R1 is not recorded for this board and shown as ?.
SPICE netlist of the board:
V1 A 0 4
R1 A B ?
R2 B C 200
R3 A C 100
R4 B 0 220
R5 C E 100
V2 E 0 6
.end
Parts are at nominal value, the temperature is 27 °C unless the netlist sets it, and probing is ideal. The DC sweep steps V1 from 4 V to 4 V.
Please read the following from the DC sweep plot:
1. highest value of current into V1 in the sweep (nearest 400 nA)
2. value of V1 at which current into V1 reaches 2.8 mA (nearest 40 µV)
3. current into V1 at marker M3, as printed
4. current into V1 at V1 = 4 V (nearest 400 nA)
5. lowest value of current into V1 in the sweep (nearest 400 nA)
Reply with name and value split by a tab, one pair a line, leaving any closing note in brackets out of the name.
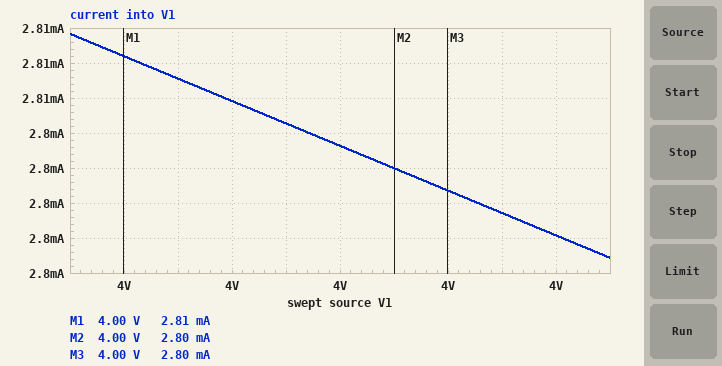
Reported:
highest value of current into V1 in the sweep	2.8096 mA
value of V1 at which current into V1 reaches 2.8 mA	3.99988 V
current into V1 at marker M3, as printed	2.80 mA
current into V1 at V1 = 4 V	2.8008 mA
lowest value of current into V1 in the sweep	2.7968 mA
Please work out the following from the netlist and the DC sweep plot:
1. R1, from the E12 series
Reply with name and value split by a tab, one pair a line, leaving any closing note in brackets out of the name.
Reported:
R1, from the E12 series	560 Ω
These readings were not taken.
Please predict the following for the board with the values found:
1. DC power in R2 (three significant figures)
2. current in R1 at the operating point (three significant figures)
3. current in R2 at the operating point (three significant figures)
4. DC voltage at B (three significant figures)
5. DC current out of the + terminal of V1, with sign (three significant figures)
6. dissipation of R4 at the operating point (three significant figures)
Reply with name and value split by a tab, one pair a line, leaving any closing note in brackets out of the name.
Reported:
DC power in R2	18.0 mW
current in R1 at the operating point	2.45 mA
current in R2 at the operating point	9.49 mA
DC voltage at B	2.63 V
DC current out of the + terminal of V1, with sign	-2.80 mA
dissipation of R4 at the operating point	31.4 mW
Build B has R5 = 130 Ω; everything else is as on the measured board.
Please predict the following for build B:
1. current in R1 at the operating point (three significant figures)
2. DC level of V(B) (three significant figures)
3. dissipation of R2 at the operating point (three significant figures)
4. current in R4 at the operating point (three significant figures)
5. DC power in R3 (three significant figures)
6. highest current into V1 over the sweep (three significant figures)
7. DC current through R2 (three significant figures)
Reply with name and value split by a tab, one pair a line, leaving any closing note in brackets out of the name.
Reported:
current in R1 at the operating point	2.58 mA
DC level of V(B)	2.55 V
dissipation of R2 at the operating point	16.3 mW
current in R4 at the operating point	11.6 mA
DC power in R3	1.29 mW
highest current into V1 over the sweep	1.02 mA
DC current through R2	9.03 mA
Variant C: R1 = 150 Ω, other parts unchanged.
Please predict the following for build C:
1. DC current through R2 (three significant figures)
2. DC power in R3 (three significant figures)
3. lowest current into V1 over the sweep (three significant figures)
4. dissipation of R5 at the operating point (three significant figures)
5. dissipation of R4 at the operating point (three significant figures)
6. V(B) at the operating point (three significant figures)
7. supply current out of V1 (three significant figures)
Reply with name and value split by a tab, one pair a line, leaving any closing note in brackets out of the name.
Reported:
DC current through R2	7.73 mA
DC power in R3	3.76 mW
lowest current into V1 over the sweep	-87.4 µA
dissipation of R5 at the operating point	19.2 mW
dissipation of R4 at the operating point	42.8 mW
V(B) at the operating point	3.07 V
supply current out of V1	79.7 µA
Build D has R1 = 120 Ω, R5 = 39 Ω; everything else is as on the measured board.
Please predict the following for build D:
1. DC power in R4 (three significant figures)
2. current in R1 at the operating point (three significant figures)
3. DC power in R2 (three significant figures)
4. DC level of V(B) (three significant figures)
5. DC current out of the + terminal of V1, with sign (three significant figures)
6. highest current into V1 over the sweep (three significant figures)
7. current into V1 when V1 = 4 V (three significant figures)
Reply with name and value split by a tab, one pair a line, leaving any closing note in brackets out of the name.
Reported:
DC power in R4	49.9 mW
current in R1 at the operating point	5.73 mA
DC power in R2	17.4 mW
DC level of V(B)	3.31 V
DC current out of the + terminal of V1, with sign	-6.04 mA
highest current into V1 over the sweep	6.05 mA
current into V1 when V1 = 4 V	6.03 mA
